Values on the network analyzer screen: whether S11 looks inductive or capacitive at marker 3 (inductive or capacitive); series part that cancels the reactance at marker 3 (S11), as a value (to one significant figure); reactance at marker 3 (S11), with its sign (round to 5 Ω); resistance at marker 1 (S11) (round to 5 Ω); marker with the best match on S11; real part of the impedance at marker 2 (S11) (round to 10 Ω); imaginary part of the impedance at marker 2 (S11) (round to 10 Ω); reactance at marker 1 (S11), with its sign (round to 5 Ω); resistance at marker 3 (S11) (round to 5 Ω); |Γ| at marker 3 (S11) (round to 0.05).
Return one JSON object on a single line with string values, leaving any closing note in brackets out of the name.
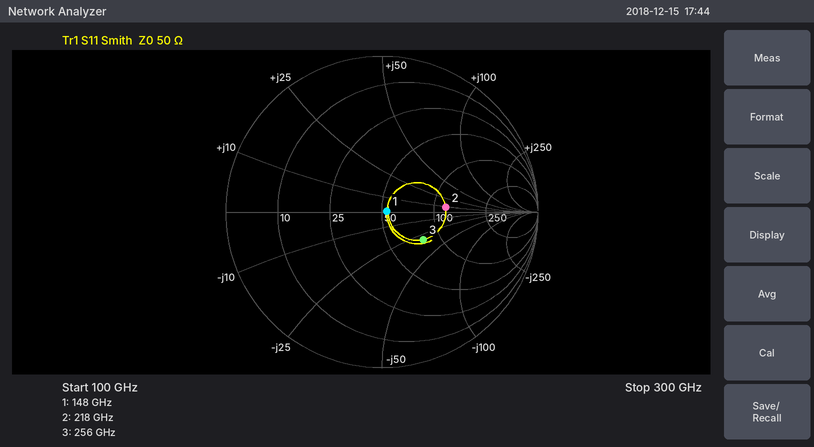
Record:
{"whether S11 looks inductive or capacitive at marker 3": "capacitive", "series part that cancels the reactance at marker 3 (S11), as a value": "20 pH", "reactance at marker 3 (S11), with its sign": "-30 Ω", "resistance at marker 1 (S11)": "55 Ω", "marker with the best match on S11": "marker 1", "real part of the impedance at marker 2 (S11)": "120 Ω", "imaginary part of the impedance at marker 2 (S11)": "+10 Ω", "reactance at marker 1 (S11), with its sign": "0 Ω", "resistance at marker 3 (S11)": "80 Ω", "|Γ| at marker 3 (S11)": "0.30"}
